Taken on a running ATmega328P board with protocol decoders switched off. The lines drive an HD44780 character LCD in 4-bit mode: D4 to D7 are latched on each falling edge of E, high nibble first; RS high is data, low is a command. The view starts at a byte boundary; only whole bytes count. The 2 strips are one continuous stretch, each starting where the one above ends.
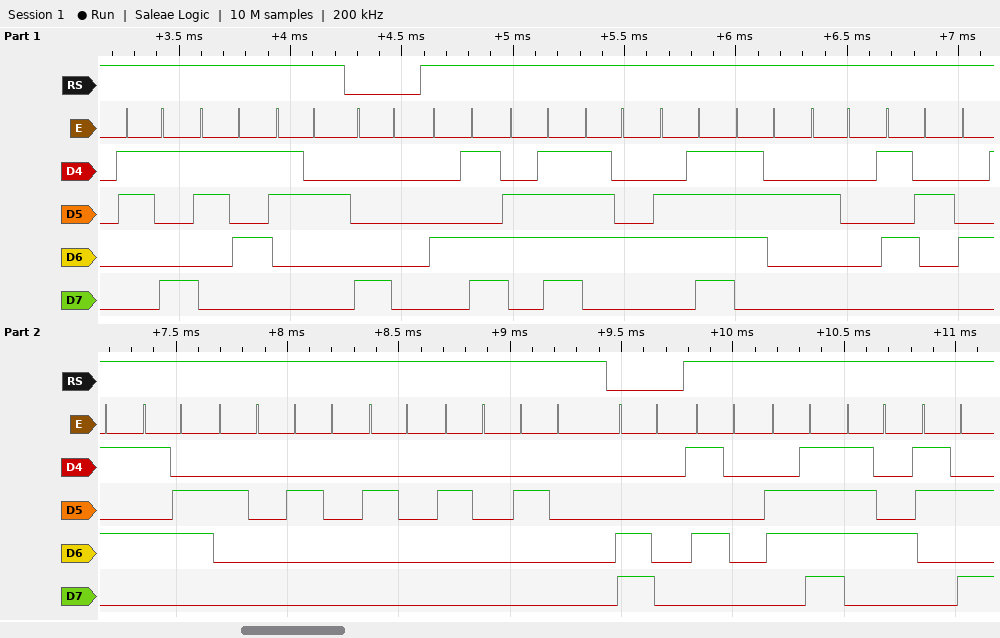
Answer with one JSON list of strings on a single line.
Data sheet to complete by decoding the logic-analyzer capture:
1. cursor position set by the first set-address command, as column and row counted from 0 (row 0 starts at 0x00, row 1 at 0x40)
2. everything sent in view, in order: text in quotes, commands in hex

["column 0, row 0", "\"952\" 0x80 \"Motor REV     \" 0xC0 \"Pot:\""]
